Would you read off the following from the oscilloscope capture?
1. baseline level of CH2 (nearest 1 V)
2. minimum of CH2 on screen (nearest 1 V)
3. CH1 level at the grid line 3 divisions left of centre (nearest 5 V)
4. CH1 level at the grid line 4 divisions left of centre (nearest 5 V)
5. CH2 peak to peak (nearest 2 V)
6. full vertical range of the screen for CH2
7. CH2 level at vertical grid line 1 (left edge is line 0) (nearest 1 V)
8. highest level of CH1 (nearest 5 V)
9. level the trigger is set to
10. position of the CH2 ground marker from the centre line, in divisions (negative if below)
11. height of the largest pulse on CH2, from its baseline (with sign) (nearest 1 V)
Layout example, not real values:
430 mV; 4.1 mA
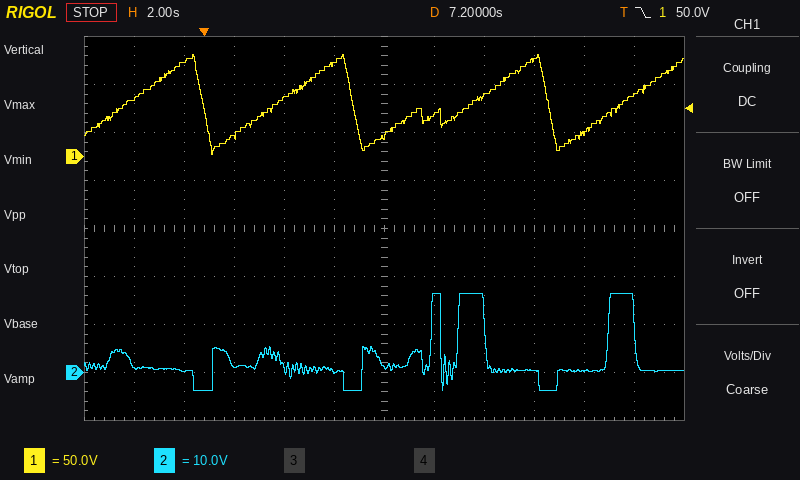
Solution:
1 V; -4 V; 20 V; 100 V; 20 V; 80 V; 1 V; 105 V; 50.0 V; -3.0 div; +16 V
